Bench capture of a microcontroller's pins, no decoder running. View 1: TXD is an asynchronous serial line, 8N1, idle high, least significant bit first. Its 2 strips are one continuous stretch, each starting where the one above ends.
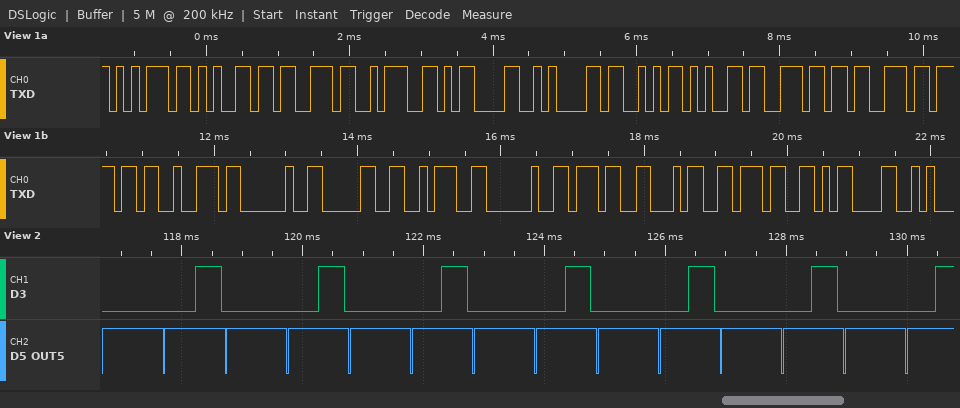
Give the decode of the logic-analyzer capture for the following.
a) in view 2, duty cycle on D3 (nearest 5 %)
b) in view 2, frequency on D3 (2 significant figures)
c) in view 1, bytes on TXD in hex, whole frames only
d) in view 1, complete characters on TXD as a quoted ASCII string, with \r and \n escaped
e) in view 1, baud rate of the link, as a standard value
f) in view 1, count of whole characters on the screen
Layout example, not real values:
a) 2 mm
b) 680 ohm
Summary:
a) 20 %
b) 490 Hz
c) 75 65 73 3A 0D 0A 53 65 6E 73 6F 72 20 30 3A 20 37 34 37 0D
d) "ues:\r\nSensor 0: 747\r"
e) 9600 baud
f) 20
